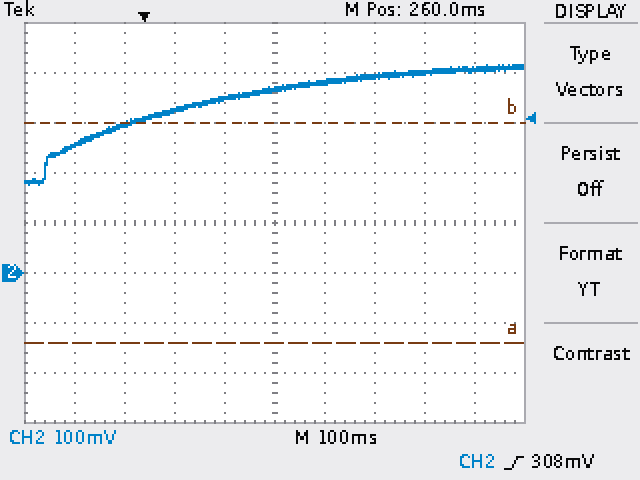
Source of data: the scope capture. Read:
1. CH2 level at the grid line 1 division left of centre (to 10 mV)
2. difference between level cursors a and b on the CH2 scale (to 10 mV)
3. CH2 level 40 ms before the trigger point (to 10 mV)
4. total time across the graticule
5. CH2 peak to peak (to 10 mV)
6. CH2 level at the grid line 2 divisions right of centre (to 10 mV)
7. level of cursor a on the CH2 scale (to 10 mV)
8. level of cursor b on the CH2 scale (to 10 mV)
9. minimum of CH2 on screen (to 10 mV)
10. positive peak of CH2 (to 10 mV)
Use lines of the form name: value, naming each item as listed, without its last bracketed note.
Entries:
CH2 level at the grid line 1 division left of centre: 350 mV
difference between level cursors a and b on the CH2 scale: 440 mV
CH2 level 40 ms before the trigger point: 300 mV
total time across the graticule: 1 s
CH2 peak to peak: 240 mV
CH2 level at the grid line 2 divisions right of centre: 390 mV
level of cursor a on the CH2 scale: -140 mV
level of cursor b on the CH2 scale: 300 mV
minimum of CH2 on screen: 180 mV
positive peak of CH2: 420 mV
